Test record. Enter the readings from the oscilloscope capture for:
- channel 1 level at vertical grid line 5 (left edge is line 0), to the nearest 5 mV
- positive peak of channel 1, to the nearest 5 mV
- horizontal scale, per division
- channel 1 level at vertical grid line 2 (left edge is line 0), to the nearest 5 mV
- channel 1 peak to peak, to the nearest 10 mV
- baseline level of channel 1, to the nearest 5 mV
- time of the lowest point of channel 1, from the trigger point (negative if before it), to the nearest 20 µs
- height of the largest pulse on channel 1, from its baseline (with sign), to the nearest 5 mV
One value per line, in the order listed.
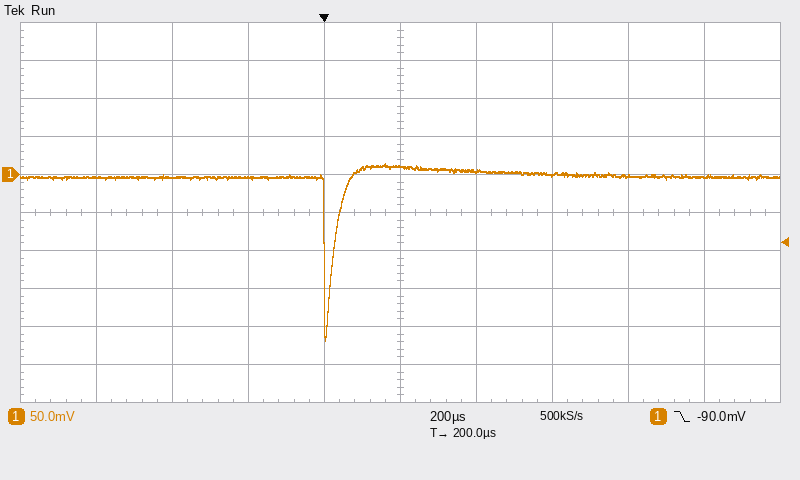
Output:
10 mV
15 mV
200 µs
-5 mV
230 mV
-5 mV
0 µs
-215 mV
